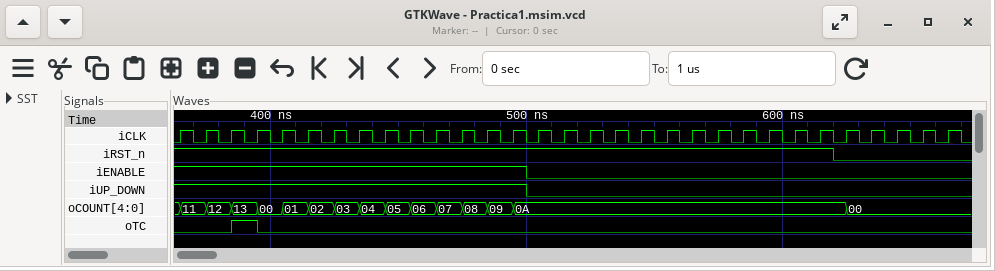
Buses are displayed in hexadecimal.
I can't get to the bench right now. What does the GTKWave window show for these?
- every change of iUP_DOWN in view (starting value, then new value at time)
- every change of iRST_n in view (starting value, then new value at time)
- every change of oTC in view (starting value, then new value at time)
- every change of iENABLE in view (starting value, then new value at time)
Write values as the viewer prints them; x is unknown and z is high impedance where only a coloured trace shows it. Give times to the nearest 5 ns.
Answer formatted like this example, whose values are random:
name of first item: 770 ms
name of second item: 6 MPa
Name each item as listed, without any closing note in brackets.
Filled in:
every change of iUP_DOWN in view: 1, 0 at 500 ns
every change of iRST_n in view: 1, 0 at 620 ns
every change of oTC in view: 0, 1 at 385 ns, 0 at 395 ns
every change of iENABLE in view: 1, 0 at 500 ns
